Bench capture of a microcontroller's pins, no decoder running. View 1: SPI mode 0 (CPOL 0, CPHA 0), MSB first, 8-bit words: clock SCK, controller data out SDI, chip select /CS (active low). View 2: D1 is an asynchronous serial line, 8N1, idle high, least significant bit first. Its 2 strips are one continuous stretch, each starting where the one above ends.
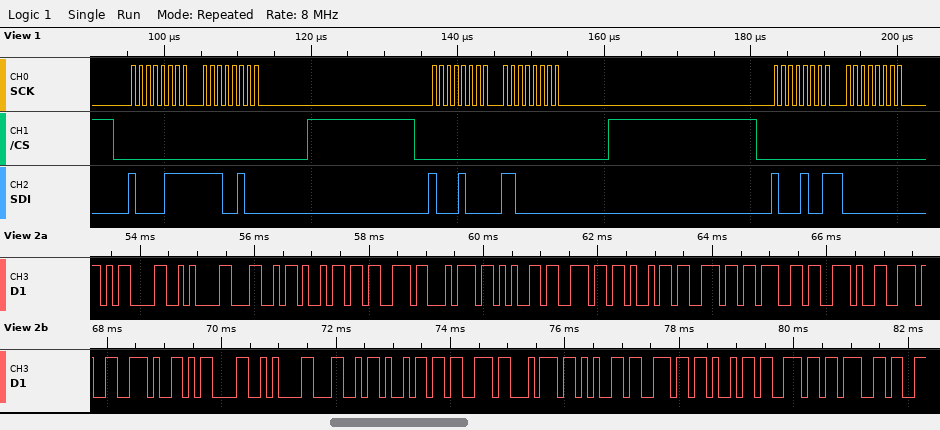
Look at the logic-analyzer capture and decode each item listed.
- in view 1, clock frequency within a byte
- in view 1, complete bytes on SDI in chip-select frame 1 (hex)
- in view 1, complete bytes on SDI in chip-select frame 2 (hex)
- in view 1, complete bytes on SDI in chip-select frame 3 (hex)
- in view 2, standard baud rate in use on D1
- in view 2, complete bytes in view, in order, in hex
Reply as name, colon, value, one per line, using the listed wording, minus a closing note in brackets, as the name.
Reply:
in view 1, clock frequency within a byte: 1 MHz
in view 1, complete bytes on SDI in chip-select frame 1: 87 E4
in view 1, complete bytes on SDI in chip-select frame 2: 88 C0
in view 1, complete bytes on SDI in chip-select frame 3: 89 00
in view 2, standard baud rate in use on D1: 9600 baud
in view 2, complete bytes in view, in order, in hex: 0x0D 0x0A 0x4C 0x69 0x73 0x74 0x65 0x6E 0x69 0x6E 0x67 0x2E 0x2E 0x2E 0x0D 0x0A 0x4C 0x69 0x73 0x74 0x65 0x6E 0x69 0x6E 0x67
